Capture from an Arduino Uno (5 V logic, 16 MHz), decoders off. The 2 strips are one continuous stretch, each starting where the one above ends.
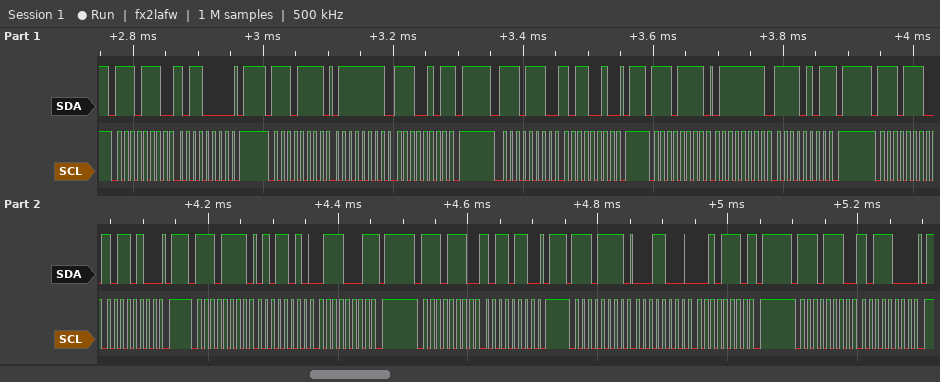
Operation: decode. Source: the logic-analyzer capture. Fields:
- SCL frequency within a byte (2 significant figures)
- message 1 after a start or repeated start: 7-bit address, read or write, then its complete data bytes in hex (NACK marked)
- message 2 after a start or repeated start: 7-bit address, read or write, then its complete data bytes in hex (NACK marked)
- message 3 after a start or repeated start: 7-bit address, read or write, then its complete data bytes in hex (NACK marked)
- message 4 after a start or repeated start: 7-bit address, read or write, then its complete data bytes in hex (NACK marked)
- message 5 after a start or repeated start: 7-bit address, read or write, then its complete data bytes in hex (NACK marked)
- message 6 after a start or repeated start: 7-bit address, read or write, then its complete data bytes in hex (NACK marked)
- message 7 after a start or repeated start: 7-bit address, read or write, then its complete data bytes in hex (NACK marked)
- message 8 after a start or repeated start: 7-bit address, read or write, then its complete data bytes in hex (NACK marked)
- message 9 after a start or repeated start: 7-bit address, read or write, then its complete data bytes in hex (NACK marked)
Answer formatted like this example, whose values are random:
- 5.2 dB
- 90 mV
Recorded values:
- 100 kHz
- 0x77 write: B0
- 0x77 read: 7F E5 NACK
- 0x77 write: B2
- 0x77 read: 7F F5 NACK
- 0x77 write: B4
- 0x77 read: 5A 71 NACK
- 0x77 write: B6
- 0x77 read: 18 2E NACK
- 0x77 write: B8
